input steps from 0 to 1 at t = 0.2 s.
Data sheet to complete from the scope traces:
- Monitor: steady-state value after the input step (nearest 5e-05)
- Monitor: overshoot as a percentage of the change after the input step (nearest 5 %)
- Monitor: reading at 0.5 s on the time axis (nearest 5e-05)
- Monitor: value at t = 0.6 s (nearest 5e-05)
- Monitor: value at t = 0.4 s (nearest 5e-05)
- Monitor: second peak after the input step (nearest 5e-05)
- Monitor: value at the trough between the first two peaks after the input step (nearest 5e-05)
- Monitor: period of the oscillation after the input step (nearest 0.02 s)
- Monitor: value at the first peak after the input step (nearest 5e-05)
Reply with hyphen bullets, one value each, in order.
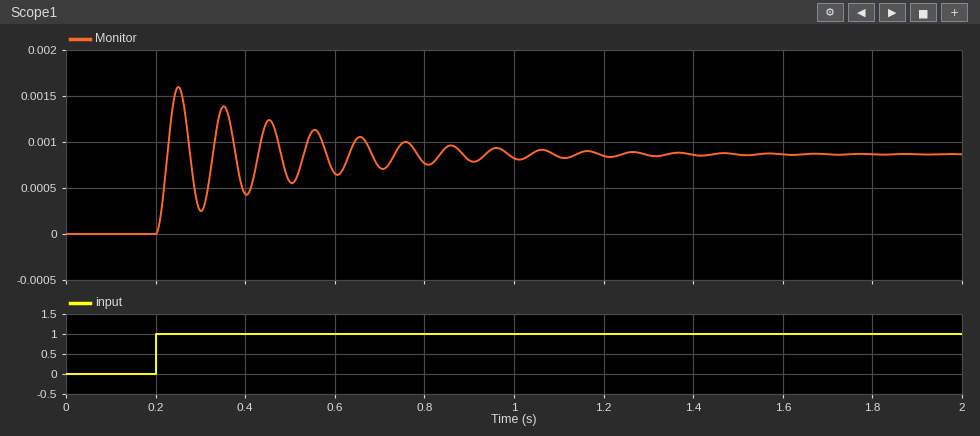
- 0.00085
- 85 %
- 0.00055
- 0.00065
- 0.00045
- 0.00140
- 0.00025
- 0.10 s
- 0.00160
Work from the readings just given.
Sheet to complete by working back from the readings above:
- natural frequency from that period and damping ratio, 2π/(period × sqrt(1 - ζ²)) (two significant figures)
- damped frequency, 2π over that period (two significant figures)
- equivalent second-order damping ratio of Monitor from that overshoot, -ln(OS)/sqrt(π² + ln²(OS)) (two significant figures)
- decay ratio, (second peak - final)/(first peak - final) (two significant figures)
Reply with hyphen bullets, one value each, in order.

- 63 rad/s
- 63 rad/s
- 0.052
- 0.73
